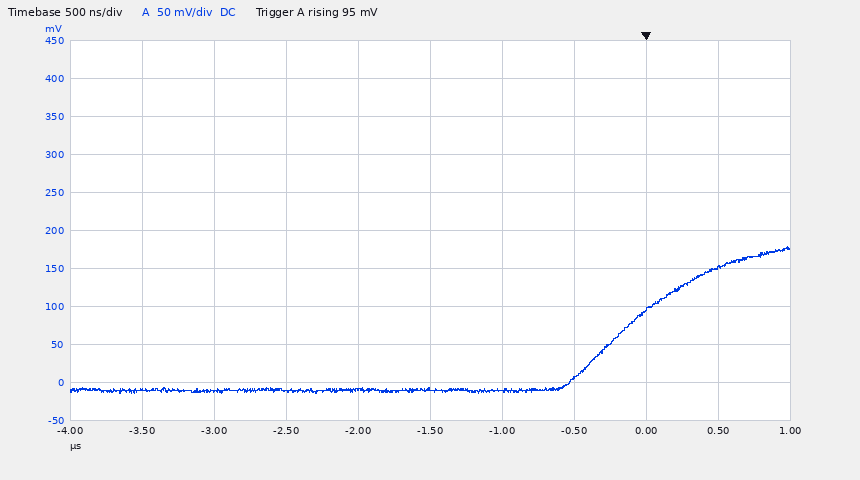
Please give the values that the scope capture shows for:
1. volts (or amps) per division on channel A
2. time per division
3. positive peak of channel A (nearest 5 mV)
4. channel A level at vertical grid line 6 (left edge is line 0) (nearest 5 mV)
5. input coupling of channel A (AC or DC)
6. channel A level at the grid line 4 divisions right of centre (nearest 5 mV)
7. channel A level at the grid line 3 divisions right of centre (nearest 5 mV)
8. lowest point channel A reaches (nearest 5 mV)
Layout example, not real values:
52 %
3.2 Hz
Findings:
50 mV
500 ns
180 mV
-10 mV
DC
150 mV
95 mV
-15 mV
